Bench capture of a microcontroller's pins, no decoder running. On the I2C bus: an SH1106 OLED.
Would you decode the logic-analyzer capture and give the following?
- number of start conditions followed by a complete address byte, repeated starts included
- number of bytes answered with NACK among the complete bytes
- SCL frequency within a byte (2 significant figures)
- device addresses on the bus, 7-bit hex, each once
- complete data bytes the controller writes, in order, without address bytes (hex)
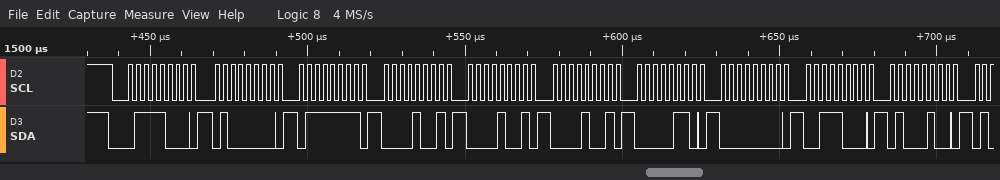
1
0
400 kHz
0x3C
40 7F 09 09 09 06 00 38 44
